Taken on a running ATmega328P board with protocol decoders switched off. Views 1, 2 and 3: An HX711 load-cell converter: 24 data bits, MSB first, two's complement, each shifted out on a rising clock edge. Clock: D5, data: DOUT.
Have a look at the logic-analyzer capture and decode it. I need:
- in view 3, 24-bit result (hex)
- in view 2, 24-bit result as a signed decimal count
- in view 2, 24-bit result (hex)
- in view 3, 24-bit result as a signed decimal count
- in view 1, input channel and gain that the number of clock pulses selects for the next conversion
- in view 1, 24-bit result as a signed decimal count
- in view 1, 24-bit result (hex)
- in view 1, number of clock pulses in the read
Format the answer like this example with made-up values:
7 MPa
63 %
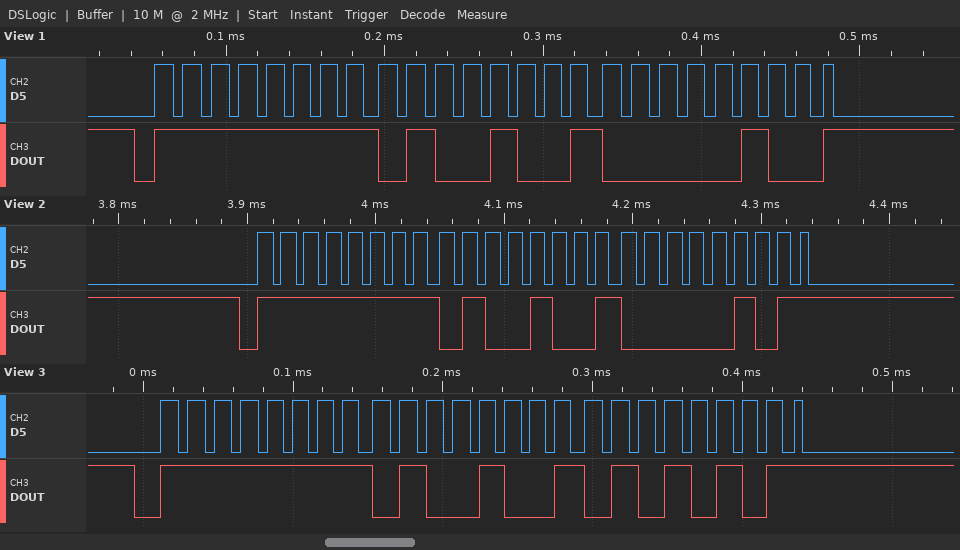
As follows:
0xFF4955
-46843
0xFF4905
-46763
channel A, gain 128
-46844
0xFF4904
25
